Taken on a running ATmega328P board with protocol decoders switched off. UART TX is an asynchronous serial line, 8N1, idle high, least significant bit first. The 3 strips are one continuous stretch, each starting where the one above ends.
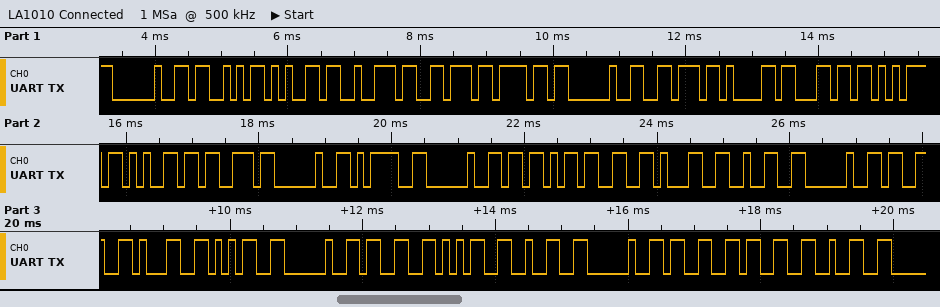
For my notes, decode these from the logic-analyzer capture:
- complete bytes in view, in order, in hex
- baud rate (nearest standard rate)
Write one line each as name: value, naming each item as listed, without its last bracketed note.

complete bytes in view, in order, in hex: 20 53 65 72 76 6F 20 76 61 6C 75 65 73 20 3D 20 5B 33 31 32 20 33 31 35 20 33 35 32 20 33 33 32
baud rate: 9600 baud
